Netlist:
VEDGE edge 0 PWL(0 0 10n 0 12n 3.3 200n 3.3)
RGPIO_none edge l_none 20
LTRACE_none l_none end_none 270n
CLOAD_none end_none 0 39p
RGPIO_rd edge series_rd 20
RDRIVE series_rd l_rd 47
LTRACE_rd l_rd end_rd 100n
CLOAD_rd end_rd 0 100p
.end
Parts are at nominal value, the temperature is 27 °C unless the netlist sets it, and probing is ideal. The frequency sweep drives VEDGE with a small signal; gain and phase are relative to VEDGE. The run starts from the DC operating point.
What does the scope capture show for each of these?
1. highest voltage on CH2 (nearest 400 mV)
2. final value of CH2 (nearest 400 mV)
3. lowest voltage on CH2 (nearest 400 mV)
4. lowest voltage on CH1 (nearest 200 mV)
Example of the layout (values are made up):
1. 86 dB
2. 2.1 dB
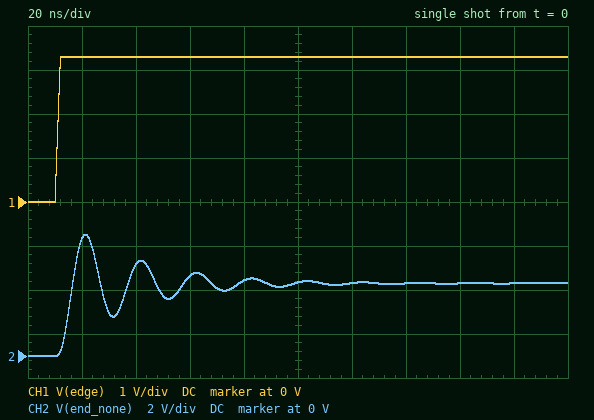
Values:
1. 5.6 V
2. 3.2 V
3. 0 V
4. 0 V
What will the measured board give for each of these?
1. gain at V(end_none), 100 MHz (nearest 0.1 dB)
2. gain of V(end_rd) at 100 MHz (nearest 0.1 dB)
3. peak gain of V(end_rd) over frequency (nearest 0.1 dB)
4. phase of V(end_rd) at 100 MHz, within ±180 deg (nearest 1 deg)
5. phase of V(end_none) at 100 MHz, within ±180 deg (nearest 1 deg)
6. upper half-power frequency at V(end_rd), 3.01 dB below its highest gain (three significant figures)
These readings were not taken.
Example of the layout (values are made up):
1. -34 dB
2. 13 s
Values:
1. -10.1 dB
2. -14.2 dB
3. 0 dB
4. -125 deg
5. -171 deg
6. 29.9 MHz
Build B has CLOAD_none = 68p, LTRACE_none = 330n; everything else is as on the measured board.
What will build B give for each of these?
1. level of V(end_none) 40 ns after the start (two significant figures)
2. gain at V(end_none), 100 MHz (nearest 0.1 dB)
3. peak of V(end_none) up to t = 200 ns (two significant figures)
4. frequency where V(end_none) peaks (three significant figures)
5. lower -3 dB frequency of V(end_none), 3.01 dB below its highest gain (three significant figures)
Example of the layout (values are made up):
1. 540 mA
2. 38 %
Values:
1. 2.0 V
2. -18.0 dB
3. 5.4 V
4. 32.9 MHz
5. 27.6 MHz
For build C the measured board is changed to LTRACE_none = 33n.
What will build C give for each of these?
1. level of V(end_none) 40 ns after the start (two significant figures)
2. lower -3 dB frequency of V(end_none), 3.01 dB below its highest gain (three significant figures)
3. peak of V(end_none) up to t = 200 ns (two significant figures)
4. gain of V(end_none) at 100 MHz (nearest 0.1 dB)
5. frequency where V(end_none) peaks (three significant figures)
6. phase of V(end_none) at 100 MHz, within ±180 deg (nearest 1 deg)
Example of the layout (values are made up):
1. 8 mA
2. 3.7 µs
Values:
1. 3.3 V
2. 48.2 MHz
3. 4.2 V
4. 3.2 dB
5. 123 MHz
6. -45 deg
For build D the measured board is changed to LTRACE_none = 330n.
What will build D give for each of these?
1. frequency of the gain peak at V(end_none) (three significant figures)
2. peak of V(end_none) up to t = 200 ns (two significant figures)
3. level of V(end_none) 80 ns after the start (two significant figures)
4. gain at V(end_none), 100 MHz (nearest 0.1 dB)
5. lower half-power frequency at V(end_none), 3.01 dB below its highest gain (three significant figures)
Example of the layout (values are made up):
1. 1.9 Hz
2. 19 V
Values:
1. 43.8 MHz
2. 5.6 V
3. 2.9 V
4. -12.3 dB
5. 38.7 MHz
